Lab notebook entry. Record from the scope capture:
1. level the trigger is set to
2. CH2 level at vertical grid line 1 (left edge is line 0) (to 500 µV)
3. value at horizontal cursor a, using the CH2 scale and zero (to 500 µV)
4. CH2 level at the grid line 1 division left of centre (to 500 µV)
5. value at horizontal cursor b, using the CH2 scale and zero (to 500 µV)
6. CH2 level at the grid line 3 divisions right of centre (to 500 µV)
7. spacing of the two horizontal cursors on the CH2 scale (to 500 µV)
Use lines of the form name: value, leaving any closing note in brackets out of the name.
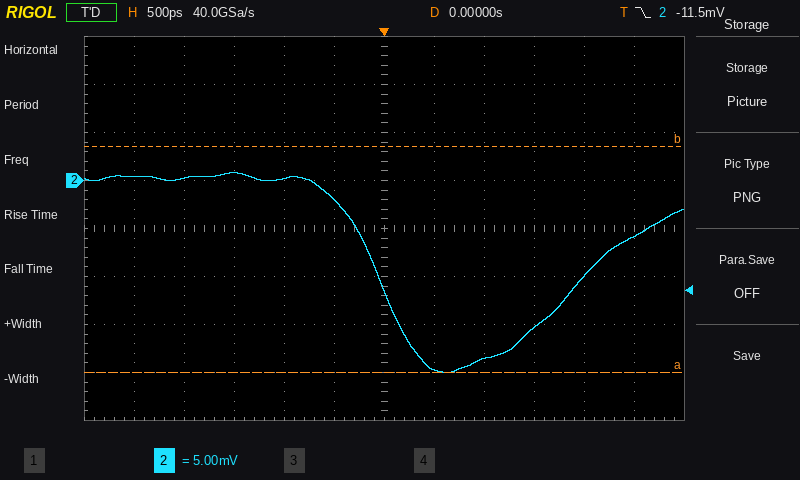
level the trigger is set to: -11.5 mV
CH2 level at vertical grid line 1 (left edge is line 0): 500 µV
value at horizontal cursor a, using the CH2 scale and zero: -20.0 mV
CH2 level at the grid line 1 division left of centre: -2.0 mV
value at horizontal cursor b, using the CH2 scale and zero: 3.5 mV
CH2 level at the grid line 3 divisions right of centre: -15.5 mV
spacing of the two horizontal cursors on the CH2 scale: 23.5 mV
